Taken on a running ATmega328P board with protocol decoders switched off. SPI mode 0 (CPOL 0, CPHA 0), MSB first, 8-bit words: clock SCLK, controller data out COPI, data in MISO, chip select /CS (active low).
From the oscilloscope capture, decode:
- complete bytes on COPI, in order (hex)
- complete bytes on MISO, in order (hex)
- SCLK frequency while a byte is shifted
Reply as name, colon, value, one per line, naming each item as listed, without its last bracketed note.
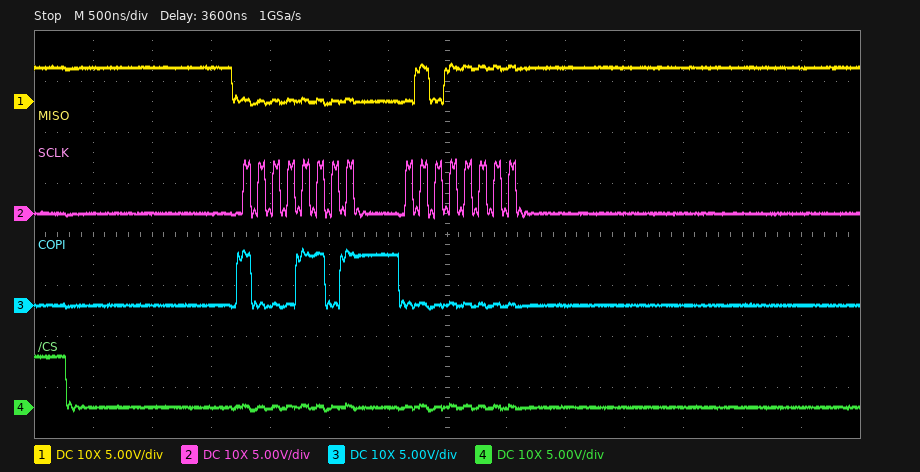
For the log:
complete bytes on COPI, in order: 0x8D 0x00
complete bytes on MISO, in order: 0x00 0x5F
SCLK frequency while a byte is shifted: 8 MHz
